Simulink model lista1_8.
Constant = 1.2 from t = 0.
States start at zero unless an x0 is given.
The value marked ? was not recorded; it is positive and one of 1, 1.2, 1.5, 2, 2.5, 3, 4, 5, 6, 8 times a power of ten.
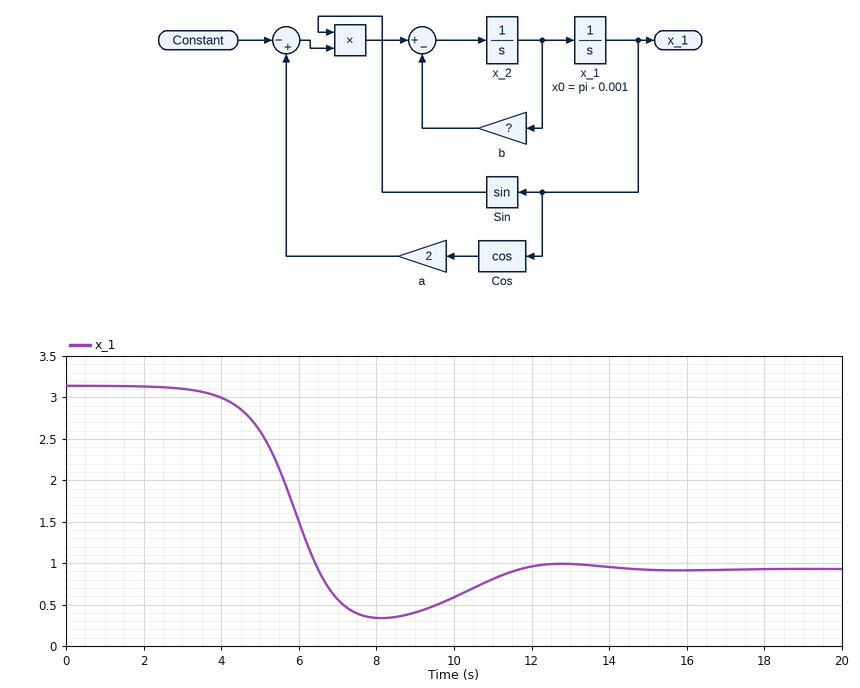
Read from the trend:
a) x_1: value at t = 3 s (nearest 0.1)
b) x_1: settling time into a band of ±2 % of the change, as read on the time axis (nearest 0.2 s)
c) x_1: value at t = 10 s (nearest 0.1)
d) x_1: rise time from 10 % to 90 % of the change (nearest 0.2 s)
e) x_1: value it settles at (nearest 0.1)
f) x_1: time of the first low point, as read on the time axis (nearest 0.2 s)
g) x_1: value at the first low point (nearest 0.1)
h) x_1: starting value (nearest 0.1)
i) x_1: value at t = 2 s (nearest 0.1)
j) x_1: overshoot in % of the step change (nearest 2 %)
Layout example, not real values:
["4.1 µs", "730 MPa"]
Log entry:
["3.1", "13.6 s", "0.6", "2.0 s", "0.9", "8.2 s", "0.3", "3.1", "3.1", "26 %"]
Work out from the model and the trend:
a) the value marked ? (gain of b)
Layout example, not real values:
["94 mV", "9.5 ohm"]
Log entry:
["1"]
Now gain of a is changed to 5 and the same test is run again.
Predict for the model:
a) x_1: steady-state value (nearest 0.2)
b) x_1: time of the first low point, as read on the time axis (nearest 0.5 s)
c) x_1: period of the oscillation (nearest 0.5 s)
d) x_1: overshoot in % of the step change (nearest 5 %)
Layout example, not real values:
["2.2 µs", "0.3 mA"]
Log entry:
["1.4", "5.0 s", "3.0 s", "35 %"]
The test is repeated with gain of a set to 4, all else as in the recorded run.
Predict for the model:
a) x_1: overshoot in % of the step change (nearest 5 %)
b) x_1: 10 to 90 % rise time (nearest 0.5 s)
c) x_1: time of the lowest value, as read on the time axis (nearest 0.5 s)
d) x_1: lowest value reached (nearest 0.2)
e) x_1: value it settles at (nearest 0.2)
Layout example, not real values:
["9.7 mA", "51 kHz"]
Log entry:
["35 %", "1.5 s", "5.5 s", "0.6", "1.2"]
